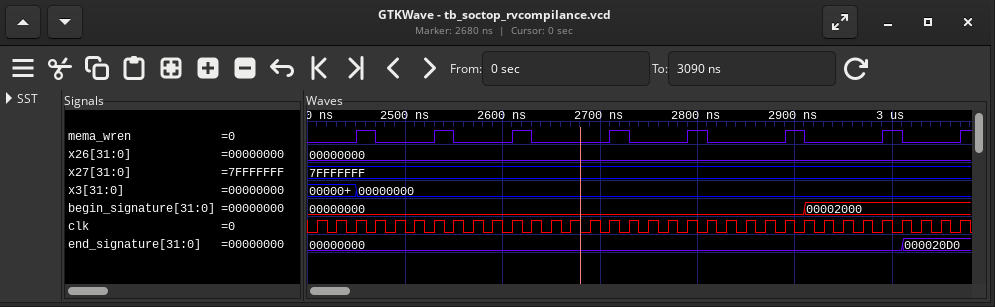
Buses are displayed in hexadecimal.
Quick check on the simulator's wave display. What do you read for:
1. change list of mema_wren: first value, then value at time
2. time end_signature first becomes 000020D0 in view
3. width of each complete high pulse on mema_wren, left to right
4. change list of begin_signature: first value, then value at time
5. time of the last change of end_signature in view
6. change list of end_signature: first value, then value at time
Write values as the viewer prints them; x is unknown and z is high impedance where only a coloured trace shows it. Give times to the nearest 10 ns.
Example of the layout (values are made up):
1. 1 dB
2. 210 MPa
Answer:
1. 0, 1 at 2450 ns, 0 at 2470 ns, 1 at 2530 ns, 0 at 2550 ns, 1 at 2610 ns, 0 at 2630 ns, 1 at 2710 ns, 0 at 2730 ns, 1 at 2790 ns, 0 at 2810 ns, 1 at 2890 ns, 0 at 2910 ns, 1 at 2990 ns, 0 at 3010 ns, 1 at 3070 ns
2. 3010 ns
3. 20 ns, 20 ns, 20 ns, 20 ns, 20 ns, 20 ns, 20 ns
4. 00000000, 00002000 at 2910 ns
5. 3010 ns
6. 00000000, 000020D0 at 3010 ns
